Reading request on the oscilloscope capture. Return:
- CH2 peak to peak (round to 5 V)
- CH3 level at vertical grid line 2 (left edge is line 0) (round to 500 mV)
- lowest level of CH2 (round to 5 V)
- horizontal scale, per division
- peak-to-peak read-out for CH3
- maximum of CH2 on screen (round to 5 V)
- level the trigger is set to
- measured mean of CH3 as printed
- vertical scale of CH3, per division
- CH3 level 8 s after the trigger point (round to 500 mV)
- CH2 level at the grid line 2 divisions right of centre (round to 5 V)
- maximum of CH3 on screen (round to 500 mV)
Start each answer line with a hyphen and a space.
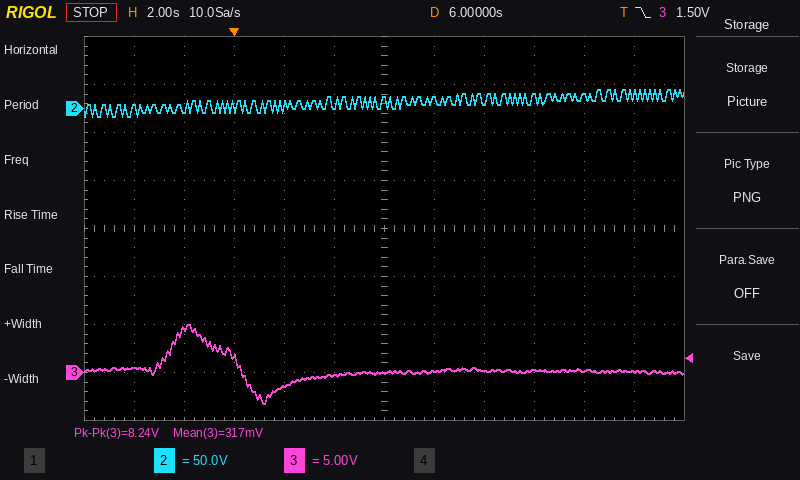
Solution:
- 30 V
- 4.5 V
- -10 V
- 2 s
- 8.24 V
- 20 V
- 1.50 V
- 317 mV
- 5 V
- 0.0 V
- 10 V
- 5.0 V
